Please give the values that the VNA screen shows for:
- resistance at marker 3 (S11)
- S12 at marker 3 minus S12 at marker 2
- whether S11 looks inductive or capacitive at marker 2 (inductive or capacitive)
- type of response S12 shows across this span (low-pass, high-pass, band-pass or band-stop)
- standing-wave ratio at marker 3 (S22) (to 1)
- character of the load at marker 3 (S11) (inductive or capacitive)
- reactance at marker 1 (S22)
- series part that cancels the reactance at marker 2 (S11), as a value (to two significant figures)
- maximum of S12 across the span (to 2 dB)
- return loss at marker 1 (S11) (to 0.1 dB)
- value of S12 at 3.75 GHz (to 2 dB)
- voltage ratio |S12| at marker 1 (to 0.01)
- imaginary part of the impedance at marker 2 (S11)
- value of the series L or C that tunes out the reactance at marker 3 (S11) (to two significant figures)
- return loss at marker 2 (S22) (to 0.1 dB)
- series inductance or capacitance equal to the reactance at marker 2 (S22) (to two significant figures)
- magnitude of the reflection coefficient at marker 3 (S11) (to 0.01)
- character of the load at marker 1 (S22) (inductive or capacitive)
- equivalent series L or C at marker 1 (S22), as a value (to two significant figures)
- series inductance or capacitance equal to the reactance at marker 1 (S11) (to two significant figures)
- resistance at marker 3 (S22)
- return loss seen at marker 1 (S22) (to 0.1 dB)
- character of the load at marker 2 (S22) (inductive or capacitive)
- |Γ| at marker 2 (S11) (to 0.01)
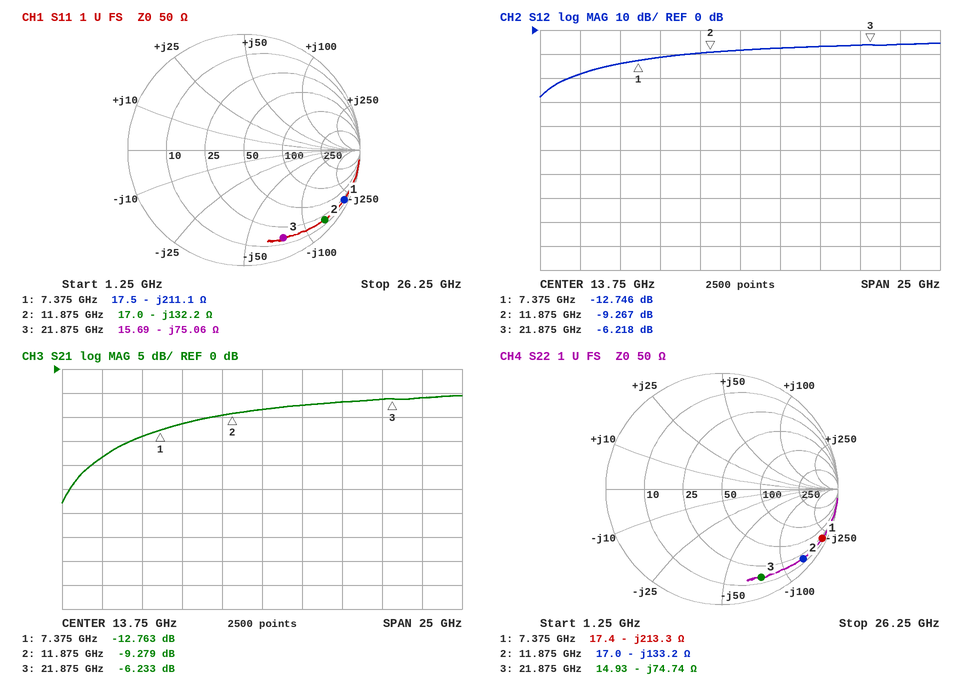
15.69 Ω
3.049 dB
capacitive
high-pass
11
capacitive
-213.3 Ω
1.8 nH
-6 dB
0.3 dB
-18 dB
0.23
-132.2 Ω
550 pH
0.7 dB
100 fF
0.83
capacitive
100 fF
100 fF
14.93 Ω
0.3 dB
capacitive
0.92
